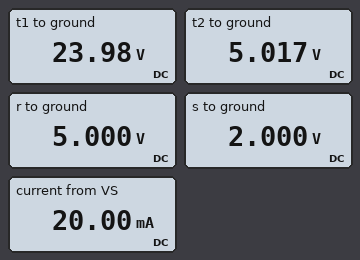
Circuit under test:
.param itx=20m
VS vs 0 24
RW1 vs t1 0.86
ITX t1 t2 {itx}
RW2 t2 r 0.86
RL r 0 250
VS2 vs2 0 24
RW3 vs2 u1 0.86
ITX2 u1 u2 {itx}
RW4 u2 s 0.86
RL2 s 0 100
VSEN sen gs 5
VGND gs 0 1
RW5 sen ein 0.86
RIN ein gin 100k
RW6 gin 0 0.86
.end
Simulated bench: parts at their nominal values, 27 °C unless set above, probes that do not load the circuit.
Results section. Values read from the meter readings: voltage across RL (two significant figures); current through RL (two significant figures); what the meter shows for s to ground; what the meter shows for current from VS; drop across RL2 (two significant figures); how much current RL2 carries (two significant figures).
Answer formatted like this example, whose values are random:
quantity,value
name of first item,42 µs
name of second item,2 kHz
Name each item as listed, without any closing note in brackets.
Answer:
quantity,value
voltage across RL,5.0 V
current through RL,20 mA
what the meter shows for s to ground,2.000 V
what the meter shows for current from VS,20.00 mA
drop across RL2,2.0 V
how much current RL2 carries,20 mA
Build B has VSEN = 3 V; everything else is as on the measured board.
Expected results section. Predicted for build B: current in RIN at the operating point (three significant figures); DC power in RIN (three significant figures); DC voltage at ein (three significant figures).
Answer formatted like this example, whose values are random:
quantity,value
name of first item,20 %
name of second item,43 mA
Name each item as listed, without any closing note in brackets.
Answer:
quantity,value
current in RIN at the operating point,40.0 µA
DC power in RIN,160 µW
DC voltage at ein,4.00 V
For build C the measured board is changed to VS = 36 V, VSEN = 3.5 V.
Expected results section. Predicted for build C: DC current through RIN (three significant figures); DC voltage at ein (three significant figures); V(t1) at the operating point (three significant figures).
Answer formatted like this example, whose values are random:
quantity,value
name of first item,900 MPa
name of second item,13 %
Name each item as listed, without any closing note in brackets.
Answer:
quantity,value
DC current through RIN,45.0 µA
DC voltage at ein,4.50 V
V(t1) at the operating point,36.0 V
